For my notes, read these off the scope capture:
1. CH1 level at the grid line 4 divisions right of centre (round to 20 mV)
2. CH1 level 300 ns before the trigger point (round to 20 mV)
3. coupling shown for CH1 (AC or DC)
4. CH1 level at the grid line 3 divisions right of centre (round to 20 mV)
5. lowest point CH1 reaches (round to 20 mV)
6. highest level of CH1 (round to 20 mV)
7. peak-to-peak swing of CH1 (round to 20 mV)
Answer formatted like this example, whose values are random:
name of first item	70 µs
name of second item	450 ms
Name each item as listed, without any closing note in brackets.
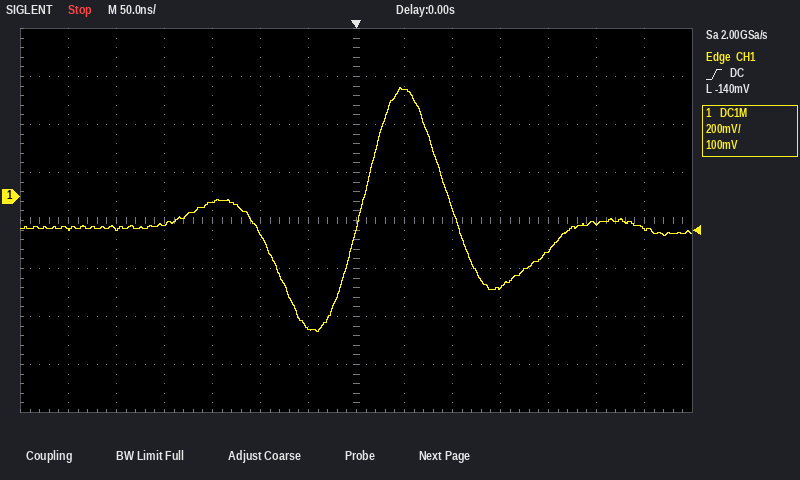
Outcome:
CH1 level at the grid line 4 divisions right of centre	-220 mV
CH1 level 300 ns before the trigger point	-140 mV
coupling shown for CH1	DC
CH1 level at the grid line 3 divisions right of centre	-380 mV
lowest point CH1 reaches	-560 mV
highest level of CH1	460 mV
peak-to-peak swing of CH1	1.02 V
